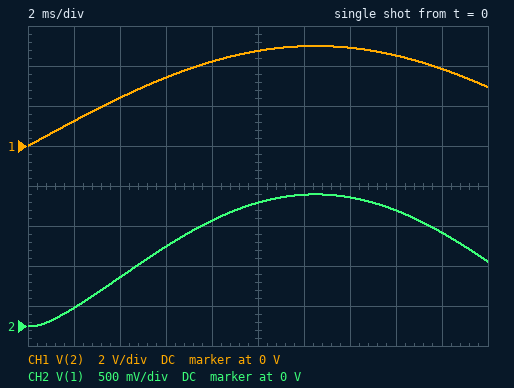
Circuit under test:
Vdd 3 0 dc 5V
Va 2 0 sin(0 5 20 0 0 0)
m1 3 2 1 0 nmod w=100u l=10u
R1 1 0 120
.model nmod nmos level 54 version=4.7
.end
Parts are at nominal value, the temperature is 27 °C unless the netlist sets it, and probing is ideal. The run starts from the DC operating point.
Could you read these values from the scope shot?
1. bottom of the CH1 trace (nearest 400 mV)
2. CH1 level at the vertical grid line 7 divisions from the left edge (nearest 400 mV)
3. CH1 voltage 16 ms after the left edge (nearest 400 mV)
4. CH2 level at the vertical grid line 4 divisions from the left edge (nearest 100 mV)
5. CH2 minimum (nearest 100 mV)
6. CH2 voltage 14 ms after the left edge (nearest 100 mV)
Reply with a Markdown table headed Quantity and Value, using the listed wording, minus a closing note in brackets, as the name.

| Quantity | Value |
|---|---|
| bottom of the CH1 trace | 0 V |
| CH1 level at the vertical grid line 7 divisions from the left edge | 4.8 V |
| CH1 voltage 16 ms after the left edge | 4.4 V |
| CH2 level at the vertical grid line 4 divisions from the left edge | 1.3 V |
| CH2 minimum | 0 V |
| CH2 voltage 14 ms after the left edge | 1.6 V |
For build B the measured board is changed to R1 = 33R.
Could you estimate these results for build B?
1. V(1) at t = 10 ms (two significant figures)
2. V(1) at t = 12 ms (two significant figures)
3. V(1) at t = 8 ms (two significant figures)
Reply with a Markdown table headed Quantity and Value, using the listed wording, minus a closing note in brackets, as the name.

| Quantity | Value |
|---|---|
| V(1) at t = 10 ms | 620 mV |
| V(1) at t = 12 ms | 660 mV |
| V(1) at t = 8 ms | 530 mV |
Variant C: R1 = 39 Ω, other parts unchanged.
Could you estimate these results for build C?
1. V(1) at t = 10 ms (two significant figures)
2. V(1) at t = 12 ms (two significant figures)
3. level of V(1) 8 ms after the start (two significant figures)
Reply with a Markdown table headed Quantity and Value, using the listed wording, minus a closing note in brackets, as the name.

| Quantity | Value |
|---|---|
| V(1) at t = 10 ms | 710 mV |
| V(1) at t = 12 ms | 760 mV |
| level of V(1) 8 ms after the start | 610 mV |
